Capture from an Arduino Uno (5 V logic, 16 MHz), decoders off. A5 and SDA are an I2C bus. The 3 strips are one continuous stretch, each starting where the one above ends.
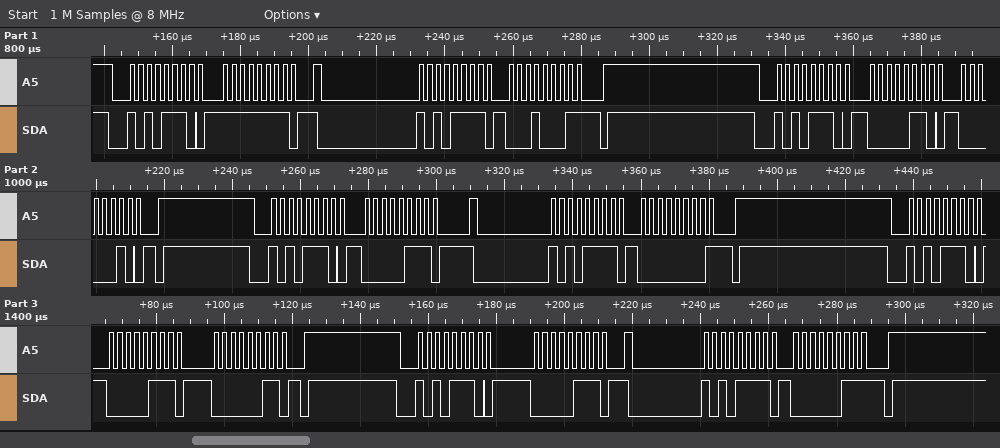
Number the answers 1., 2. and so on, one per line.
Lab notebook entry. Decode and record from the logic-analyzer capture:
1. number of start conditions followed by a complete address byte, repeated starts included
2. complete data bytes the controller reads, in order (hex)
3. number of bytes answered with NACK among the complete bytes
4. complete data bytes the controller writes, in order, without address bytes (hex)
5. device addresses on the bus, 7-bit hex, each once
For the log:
1. 8
2. 11 00 03
3. 3
4. FF 06 02 07 07 03 07
5. 0x57
